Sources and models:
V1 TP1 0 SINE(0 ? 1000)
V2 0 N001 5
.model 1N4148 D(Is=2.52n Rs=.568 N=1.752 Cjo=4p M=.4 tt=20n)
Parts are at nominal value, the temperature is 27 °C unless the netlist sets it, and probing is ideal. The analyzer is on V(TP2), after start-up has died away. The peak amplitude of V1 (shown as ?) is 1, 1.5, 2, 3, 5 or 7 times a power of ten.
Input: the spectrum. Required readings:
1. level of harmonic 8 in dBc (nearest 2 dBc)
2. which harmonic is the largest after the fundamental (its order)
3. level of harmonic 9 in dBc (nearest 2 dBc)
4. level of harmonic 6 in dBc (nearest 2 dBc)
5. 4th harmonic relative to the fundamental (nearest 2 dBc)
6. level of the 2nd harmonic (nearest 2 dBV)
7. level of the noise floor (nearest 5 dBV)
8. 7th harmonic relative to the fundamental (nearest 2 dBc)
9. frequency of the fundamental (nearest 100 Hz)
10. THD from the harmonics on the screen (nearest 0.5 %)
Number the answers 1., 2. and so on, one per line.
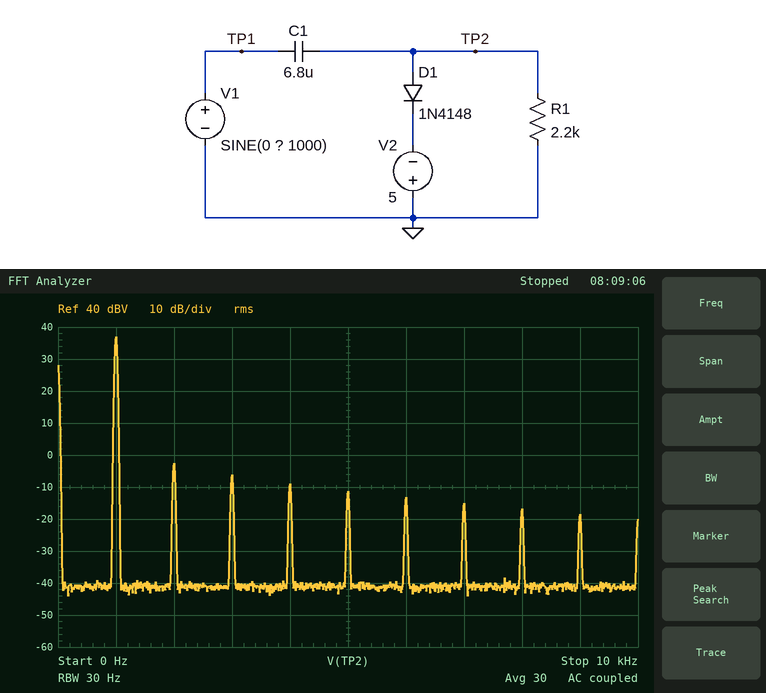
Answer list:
1. -54 dBc
2. 2
3. -56 dBc
4. -50 dBc
5. -46 dBc
6. -2 dBV
7. -40 dBV
8. -52 dBc
9. 1.0 kHz
10. 1.5 %
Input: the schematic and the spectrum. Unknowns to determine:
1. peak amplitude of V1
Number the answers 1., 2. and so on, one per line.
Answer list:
1. 100 V
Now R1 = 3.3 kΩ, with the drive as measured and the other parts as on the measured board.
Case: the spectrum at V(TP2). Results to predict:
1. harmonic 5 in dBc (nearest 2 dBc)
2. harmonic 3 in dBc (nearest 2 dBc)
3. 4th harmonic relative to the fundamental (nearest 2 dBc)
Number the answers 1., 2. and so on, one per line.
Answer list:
1. -52 dBc
2. -46 dBc
3. -50 dBc
